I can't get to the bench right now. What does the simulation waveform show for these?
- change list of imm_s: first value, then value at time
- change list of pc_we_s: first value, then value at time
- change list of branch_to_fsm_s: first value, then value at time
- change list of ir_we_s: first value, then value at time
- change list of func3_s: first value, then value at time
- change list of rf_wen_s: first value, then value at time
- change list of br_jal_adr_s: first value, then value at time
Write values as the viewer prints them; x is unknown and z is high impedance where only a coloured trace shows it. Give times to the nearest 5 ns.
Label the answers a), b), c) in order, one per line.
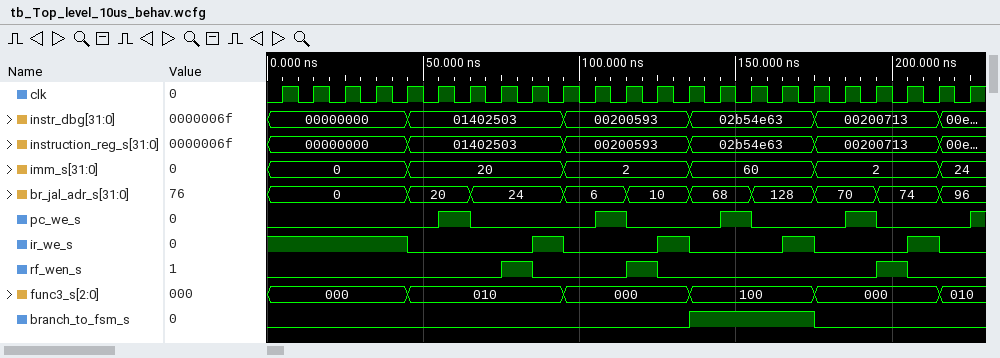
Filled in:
a) 0, 20 at 45 ns, 2 at 95 ns, 60 at 135 ns, 2 at 175 ns, 24 at 215 ns
b) 0, 1 at 55 ns, 0 at 65 ns, 1 at 105 ns, 0 at 115 ns, 1 at 145 ns, 0 at 155 ns, 1 at 185 ns, 0 at 195 ns, 1 at 225 ns
c) 0, 1 at 135 ns, 0 at 175 ns
d) 1, 0 at 45 ns, 1 at 85 ns, 0 at 95 ns, 1 at 125 ns, 0 at 135 ns, 1 at 165 ns, 0 at 175 ns, 1 at 205 ns, 0 at 215 ns
e) 000, 010 at 45 ns, 000 at 95 ns, 100 at 135 ns, 000 at 175 ns, 010 at 215 ns
f) 0, 1 at 75 ns, 0 at 85 ns, 1 at 115 ns, 0 at 125 ns, 1 at 195 ns, 0 at 205 ns
g) 0, 20 at 45 ns, 24 at 65 ns, 6 at 95 ns, 10 at 115 ns, 68 at 135 ns, 128 at 155 ns, 70 at 175 ns, 74 at 195 ns, 96 at 215 ns
